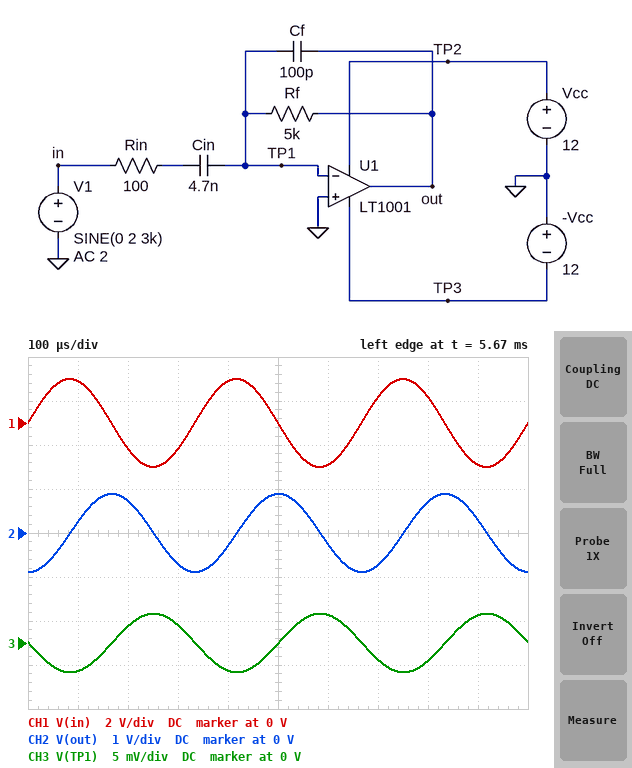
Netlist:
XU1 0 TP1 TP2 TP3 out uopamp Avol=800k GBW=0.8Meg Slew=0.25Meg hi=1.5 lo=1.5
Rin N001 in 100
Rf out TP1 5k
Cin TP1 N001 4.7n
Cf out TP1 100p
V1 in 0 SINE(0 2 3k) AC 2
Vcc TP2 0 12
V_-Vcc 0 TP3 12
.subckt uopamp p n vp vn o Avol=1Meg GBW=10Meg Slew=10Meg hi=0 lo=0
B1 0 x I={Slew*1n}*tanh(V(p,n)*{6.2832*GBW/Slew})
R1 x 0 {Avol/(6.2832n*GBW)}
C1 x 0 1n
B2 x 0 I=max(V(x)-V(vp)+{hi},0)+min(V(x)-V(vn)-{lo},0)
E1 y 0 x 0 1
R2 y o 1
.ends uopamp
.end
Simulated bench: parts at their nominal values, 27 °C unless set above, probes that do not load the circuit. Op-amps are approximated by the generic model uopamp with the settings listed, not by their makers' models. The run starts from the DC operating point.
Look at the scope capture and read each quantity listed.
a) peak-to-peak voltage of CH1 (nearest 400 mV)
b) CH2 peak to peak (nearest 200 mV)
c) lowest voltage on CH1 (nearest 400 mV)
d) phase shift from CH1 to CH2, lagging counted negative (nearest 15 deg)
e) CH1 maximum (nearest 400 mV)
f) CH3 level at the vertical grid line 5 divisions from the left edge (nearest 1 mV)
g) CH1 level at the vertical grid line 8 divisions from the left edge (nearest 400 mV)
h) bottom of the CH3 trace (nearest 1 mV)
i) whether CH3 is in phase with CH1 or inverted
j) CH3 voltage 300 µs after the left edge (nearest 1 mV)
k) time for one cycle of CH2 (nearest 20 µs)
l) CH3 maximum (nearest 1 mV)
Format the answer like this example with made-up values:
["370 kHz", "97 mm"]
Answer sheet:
["4.0 V", "1.8 V", "-2.0 V", "-90 deg", "2.0 V", "0 V", "1.2 V", "-3 mV", "inverted", "2 mV", "340 µs", "3 mV"]
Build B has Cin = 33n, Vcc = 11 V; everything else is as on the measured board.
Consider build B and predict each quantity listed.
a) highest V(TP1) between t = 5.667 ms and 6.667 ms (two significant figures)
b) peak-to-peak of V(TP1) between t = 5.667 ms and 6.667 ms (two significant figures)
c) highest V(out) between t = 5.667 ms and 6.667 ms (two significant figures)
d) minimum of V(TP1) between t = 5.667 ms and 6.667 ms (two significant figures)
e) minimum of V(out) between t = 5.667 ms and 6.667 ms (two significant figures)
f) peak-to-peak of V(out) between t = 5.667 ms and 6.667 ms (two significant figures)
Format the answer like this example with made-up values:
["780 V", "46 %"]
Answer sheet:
["26 mV", "51 mV", "6.3 V", "-26 mV", "-6.3 V", "13 V"]
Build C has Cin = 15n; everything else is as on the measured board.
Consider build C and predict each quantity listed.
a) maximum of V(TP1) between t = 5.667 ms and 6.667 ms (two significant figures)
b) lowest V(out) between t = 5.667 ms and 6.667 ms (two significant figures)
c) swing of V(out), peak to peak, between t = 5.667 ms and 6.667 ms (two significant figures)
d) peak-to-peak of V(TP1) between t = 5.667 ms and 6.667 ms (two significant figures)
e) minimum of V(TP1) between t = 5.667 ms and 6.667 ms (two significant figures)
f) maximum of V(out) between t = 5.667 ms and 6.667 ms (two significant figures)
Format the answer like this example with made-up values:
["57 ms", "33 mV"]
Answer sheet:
["11 mV", "-2.8 V", "5.7 V", "22 mV", "-11 mV", "2.8 V"]
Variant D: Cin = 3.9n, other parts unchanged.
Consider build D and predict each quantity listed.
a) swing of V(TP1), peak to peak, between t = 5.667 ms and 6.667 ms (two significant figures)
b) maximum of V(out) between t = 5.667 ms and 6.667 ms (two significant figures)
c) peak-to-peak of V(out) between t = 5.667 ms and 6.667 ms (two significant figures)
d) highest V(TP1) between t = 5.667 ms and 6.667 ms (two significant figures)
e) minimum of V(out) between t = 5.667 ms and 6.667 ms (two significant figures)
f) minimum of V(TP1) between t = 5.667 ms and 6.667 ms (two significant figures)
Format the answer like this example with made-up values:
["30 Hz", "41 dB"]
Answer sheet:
["5.5 mV", "740 mV", "1.5 V", "2.8 mV", "-740 mV", "-2.8 mV"]
